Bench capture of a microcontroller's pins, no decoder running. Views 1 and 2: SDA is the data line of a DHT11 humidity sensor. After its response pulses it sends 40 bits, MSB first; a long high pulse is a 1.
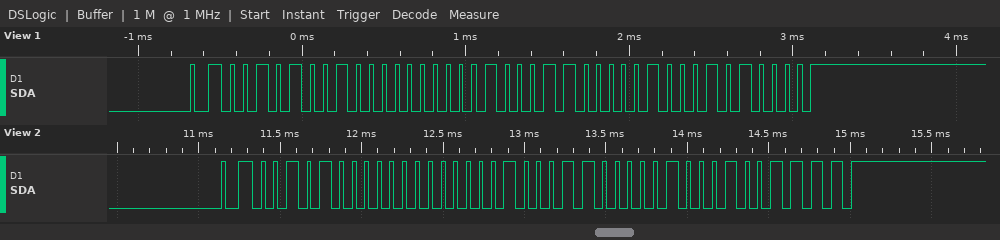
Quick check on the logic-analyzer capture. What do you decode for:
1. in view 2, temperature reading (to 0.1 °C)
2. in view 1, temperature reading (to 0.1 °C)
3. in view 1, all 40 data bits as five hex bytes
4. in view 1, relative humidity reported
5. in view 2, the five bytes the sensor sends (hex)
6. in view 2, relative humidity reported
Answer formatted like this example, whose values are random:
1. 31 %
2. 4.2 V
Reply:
1. 35.4 °C
2. 35.4 °C
3. 29 00 23 04 50
4. 41 %
5. 28 00 23 04 4F
6. 40 %
